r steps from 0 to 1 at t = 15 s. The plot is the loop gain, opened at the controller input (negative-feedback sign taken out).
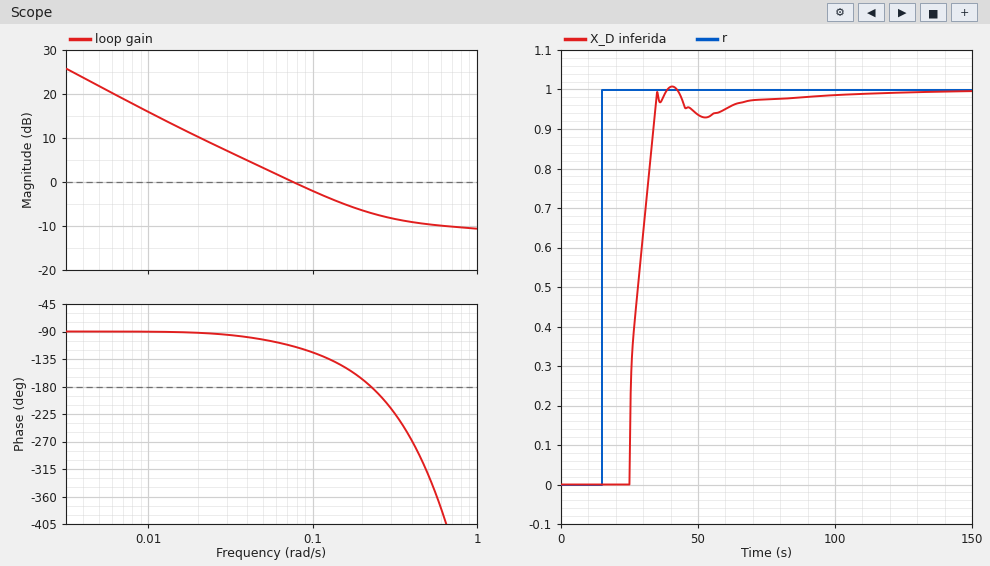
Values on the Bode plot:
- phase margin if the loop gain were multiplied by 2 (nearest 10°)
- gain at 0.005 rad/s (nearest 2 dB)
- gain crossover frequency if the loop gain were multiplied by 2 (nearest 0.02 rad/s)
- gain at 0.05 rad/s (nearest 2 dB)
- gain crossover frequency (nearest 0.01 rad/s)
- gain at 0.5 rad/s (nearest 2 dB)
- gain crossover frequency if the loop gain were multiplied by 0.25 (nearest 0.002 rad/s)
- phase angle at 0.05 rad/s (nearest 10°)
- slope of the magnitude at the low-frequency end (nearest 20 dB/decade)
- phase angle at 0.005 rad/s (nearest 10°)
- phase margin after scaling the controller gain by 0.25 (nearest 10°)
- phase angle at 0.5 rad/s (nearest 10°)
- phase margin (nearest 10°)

20°
22 dB
0.18 rad/s
4 dB
0.08 rad/s
-10 dB
0.016 rad/s
-100°
-20 dB/decade
-90°
90°
-320°
70°
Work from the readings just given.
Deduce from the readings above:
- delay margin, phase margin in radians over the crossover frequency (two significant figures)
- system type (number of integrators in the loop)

15 s
1
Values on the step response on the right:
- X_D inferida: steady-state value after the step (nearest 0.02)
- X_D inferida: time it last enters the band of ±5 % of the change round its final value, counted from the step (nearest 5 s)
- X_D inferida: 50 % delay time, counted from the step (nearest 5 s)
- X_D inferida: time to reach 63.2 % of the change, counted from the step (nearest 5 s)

1.00
45 s
15 s
15 s
